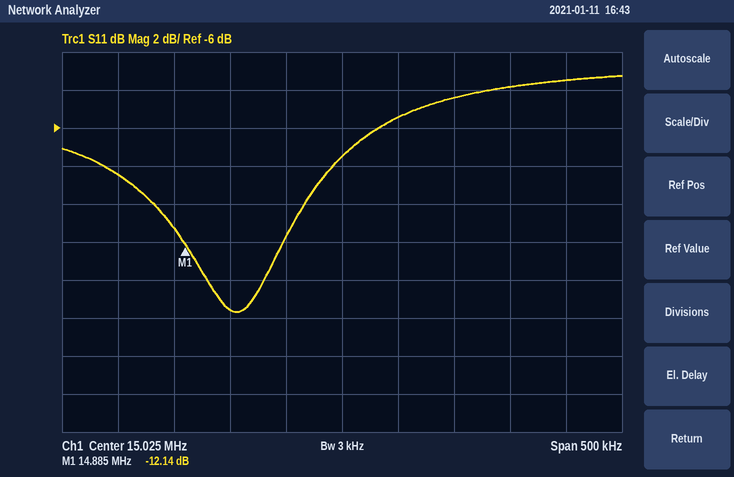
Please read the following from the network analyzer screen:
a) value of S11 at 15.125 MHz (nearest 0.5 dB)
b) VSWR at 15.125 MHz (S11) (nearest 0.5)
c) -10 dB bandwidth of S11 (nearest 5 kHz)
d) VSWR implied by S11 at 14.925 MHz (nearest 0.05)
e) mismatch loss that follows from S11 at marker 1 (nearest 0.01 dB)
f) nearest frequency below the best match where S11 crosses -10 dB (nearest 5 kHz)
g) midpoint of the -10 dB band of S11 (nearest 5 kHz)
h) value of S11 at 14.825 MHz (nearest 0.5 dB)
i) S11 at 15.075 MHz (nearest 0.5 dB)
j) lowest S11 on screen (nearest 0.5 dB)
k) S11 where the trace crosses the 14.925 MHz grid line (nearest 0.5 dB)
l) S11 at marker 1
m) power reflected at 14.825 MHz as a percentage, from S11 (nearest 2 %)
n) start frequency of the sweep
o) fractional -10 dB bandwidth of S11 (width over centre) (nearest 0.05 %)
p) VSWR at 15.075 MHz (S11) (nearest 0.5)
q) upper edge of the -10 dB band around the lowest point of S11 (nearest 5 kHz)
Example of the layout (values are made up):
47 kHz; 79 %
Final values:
-4.5 dB; 4.0; 135 kHz; 1.40; 0.27 dB; 14.855 MHz; 14.925 MHz; -8.5 dB; -5.5 dB; -15.5 dB; -15.5 dB; -12.14 dB; 14 %; 14.775 MHz; 0.90 %; 3.5; 14.990 MHz
